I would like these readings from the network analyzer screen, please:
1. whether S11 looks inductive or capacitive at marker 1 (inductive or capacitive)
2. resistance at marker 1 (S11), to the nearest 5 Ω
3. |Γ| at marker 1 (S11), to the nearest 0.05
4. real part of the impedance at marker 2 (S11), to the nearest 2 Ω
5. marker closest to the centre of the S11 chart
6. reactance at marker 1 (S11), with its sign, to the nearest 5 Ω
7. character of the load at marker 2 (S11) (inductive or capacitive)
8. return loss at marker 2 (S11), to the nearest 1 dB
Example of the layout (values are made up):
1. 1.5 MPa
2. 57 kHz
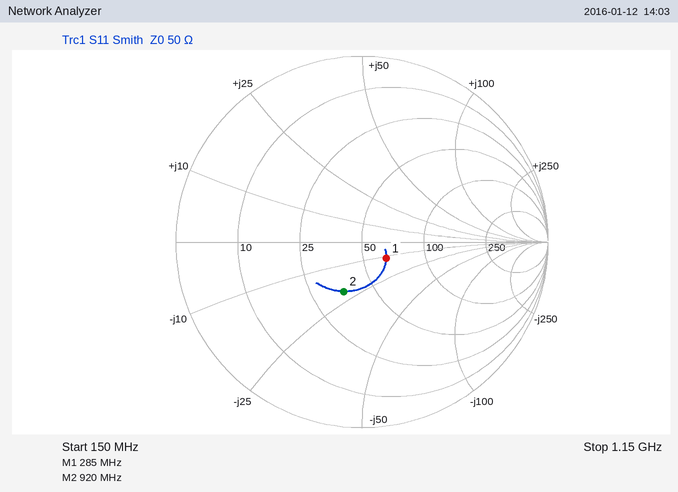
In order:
1. capacitive
2. 65 Ω
3. 0.15
4. 36 Ω
5. marker 1
6. -10 Ω
7. capacitive
8. 11 dB
